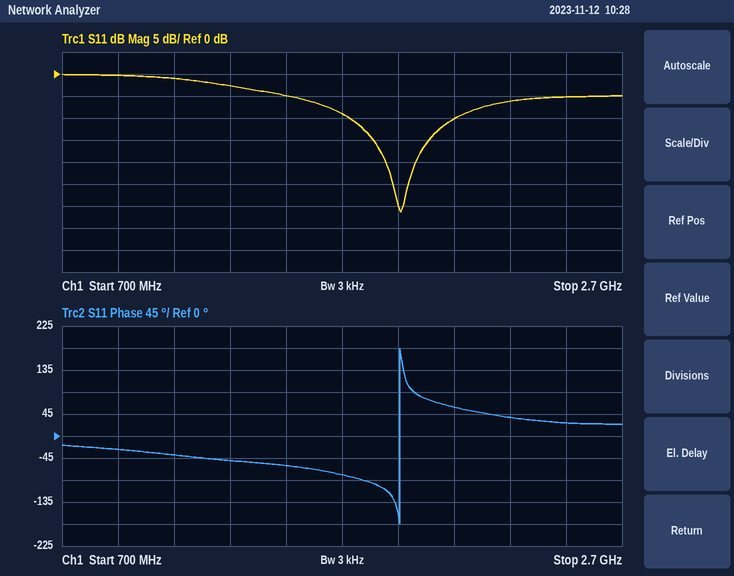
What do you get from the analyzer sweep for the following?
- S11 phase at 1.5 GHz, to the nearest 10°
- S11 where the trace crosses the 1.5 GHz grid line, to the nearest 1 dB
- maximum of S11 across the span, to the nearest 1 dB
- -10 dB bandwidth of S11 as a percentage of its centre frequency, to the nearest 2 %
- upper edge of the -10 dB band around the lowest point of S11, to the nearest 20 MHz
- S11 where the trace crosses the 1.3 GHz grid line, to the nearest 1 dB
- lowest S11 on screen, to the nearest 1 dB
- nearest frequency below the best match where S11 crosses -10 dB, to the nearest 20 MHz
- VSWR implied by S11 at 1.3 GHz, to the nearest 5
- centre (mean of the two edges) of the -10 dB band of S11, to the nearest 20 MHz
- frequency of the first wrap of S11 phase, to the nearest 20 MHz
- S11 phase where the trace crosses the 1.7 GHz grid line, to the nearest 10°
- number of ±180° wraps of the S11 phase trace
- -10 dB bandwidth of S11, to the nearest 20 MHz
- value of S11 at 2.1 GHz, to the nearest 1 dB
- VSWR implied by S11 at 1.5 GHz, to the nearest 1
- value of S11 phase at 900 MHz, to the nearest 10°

-60°
-5 dB
0 dB
20 %
2.10 GHz
-3 dB
-31 dB
1.72 GHz
5
1.92 GHz
1.90 GHz
-80°
1
380 MHz
-10 dB
4
-30°
